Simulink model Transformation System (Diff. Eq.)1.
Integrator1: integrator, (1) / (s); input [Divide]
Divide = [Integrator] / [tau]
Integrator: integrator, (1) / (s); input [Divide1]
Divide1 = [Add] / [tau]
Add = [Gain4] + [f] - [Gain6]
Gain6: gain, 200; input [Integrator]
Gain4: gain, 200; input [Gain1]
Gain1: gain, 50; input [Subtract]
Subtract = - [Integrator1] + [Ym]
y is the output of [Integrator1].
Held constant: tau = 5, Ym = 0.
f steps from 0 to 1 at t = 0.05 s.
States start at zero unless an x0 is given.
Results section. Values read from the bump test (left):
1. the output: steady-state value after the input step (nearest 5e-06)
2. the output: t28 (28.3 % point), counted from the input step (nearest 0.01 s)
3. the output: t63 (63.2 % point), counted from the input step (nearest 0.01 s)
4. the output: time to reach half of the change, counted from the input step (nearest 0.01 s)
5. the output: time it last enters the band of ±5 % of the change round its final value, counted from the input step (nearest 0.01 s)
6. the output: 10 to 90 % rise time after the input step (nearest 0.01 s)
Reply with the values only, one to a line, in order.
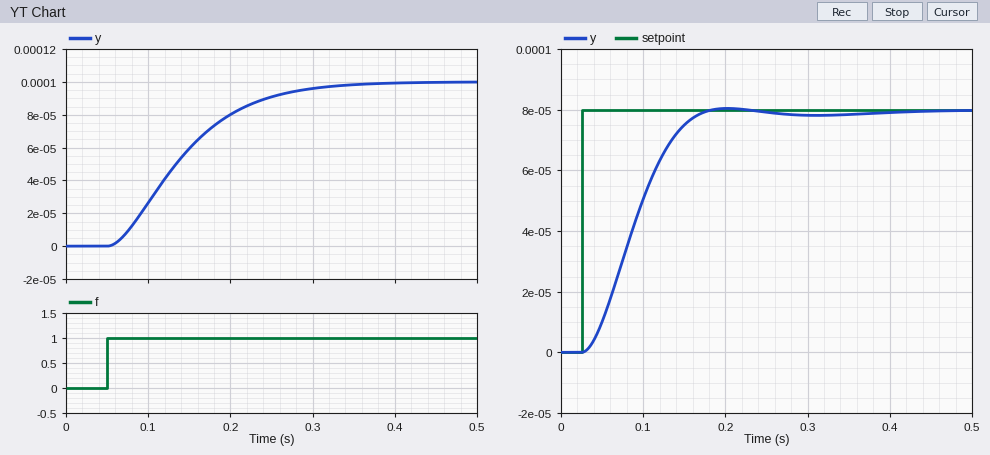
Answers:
0.000100
0.05 s
0.11 s
0.08 s
0.24 s
0.17 s
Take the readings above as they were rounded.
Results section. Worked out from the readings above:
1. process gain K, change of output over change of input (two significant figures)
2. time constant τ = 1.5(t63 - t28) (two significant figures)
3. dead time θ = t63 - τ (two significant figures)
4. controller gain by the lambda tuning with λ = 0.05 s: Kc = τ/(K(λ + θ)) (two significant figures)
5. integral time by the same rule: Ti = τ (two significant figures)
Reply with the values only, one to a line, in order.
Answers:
0.00010
0.090 s
0.020 s
13000
0.090 s
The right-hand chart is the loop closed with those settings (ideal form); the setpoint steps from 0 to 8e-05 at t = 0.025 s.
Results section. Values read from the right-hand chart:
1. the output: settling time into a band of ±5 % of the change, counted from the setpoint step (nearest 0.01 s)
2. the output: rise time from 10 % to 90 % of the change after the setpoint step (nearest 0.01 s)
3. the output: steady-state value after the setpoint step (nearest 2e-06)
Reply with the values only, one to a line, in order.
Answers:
0.13 s
0.09 s
0.000080
